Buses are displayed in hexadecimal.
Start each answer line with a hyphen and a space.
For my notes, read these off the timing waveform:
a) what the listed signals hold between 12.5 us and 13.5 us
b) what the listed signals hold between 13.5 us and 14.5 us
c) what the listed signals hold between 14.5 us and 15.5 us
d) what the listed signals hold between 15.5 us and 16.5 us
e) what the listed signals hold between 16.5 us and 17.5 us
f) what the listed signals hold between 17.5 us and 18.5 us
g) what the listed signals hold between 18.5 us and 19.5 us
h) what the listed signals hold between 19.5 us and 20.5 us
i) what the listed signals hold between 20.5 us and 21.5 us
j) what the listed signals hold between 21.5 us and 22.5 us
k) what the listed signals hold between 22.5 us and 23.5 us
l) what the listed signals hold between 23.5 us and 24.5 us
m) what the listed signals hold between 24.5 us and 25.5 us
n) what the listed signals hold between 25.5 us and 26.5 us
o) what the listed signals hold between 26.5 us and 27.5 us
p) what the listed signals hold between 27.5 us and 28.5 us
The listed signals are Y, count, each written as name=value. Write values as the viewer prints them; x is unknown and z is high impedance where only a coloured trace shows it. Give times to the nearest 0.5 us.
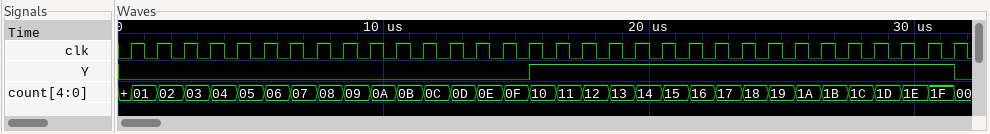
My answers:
- Y=0, count=0D
- Y=0, count=0E
- Y=0, count=0F
- Y=1, count=10
- Y=1, count=11
- Y=1, count=12
- Y=1, count=13
- Y=1, count=14
- Y=1, count=15
- Y=1, count=16
- Y=1, count=17
- Y=1, count=18
- Y=1, count=19
- Y=1, count=1A
- Y=1, count=1B
- Y=1, count=1C
